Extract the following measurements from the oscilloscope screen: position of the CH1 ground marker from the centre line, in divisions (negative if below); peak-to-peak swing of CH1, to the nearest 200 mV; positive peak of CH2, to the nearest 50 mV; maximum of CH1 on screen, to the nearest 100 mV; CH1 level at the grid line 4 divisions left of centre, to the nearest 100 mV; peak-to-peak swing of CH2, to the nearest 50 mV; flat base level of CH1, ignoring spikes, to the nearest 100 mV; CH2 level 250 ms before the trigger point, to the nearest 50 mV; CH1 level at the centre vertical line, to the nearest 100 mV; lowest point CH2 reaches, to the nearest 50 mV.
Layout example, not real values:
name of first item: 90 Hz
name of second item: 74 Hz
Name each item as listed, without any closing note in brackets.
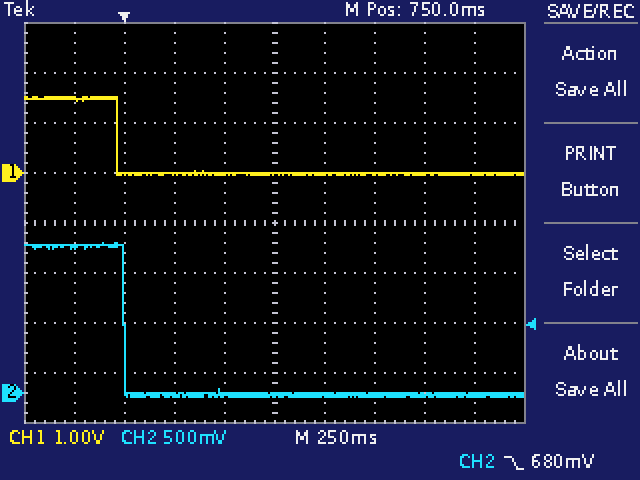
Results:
position of the CH1 ground marker from the centre line, in divisions: +1.0 div
peak-to-peak swing of CH1, to the nearest 200 mV: 1.6 V
positive peak of CH2, to the nearest 50 mV: 1.50 V
maximum of CH1 on screen, to the nearest 100 mV: 1.5 V
CH1 level at the grid line 4 divisions left of centre, to the nearest 100 mV: 1.5 V
peak-to-peak swing of CH2, to the nearest 50 mV: 1.55 V
flat base level of CH1, ignoring spikes, to the nearest 100 mV: 0.0 V
CH2 level 250 ms before the trigger point, to the nearest 50 mV: 1.45 V
CH1 level at the centre vertical line, to the nearest 100 mV: 0.0 V
lowest point CH2 reaches, to the nearest 50 mV: -50 mV
